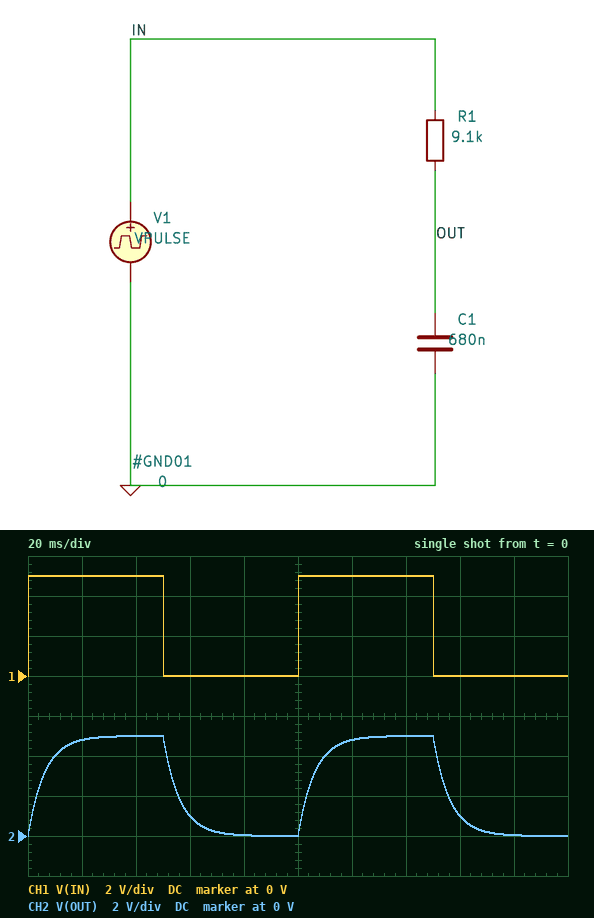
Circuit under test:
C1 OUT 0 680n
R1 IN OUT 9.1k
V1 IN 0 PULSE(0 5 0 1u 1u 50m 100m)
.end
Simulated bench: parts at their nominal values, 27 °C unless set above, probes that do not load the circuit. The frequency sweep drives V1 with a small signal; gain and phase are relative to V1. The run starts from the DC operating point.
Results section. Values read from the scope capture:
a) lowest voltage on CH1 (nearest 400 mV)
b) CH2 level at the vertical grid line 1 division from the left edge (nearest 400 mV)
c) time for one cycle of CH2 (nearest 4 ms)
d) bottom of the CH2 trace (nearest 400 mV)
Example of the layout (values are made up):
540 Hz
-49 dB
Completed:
0 V
4.8 V
100 ms
0 V
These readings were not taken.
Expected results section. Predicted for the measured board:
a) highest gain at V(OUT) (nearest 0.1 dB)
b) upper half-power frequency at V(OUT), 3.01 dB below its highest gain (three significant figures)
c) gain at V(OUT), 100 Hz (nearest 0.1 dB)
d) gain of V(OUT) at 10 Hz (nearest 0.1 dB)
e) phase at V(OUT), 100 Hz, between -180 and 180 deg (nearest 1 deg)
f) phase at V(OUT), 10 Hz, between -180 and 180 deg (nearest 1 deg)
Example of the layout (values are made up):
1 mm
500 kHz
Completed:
0 dB
25.7 Hz
-12.1 dB
-0.6 dB
-76 deg
-21 deg
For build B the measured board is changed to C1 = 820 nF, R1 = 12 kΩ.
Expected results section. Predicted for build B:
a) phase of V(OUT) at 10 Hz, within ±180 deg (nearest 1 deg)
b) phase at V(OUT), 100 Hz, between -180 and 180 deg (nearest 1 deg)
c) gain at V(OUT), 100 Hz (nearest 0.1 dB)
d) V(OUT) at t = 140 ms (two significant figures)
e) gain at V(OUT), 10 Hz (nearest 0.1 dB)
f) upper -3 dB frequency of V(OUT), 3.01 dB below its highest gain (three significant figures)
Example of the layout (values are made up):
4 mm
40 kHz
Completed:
-32 deg
-81 deg
-15.9 dB
4.9 V
-1.4 dB
16.2 Hz
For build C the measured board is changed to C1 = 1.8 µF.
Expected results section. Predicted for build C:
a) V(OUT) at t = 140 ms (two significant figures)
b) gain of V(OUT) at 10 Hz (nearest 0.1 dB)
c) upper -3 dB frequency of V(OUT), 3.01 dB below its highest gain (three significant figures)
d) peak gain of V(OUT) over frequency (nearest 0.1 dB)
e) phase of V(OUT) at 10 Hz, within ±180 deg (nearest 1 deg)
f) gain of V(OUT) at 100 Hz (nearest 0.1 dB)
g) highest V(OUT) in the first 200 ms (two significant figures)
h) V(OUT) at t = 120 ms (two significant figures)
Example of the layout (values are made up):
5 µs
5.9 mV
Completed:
4.6 V
-3.1 dB
9.72 Hz
0 dB
-46 deg
-20.3 dB
4.8 V
3.6 V
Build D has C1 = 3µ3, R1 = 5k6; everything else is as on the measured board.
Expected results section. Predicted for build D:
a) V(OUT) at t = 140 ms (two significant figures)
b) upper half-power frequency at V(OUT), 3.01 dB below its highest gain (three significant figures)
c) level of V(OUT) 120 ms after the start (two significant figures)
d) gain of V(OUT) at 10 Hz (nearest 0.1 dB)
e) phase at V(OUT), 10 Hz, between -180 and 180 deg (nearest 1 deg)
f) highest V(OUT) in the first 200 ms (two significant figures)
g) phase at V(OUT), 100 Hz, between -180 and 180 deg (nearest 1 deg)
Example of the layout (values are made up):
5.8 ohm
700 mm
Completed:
4.5 V
8.61 Hz
3.4 V
-3.7 dB
-49 deg
4.7 V
-85 deg
